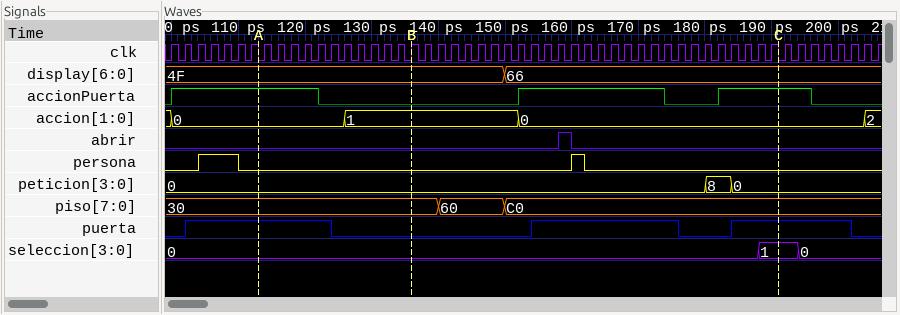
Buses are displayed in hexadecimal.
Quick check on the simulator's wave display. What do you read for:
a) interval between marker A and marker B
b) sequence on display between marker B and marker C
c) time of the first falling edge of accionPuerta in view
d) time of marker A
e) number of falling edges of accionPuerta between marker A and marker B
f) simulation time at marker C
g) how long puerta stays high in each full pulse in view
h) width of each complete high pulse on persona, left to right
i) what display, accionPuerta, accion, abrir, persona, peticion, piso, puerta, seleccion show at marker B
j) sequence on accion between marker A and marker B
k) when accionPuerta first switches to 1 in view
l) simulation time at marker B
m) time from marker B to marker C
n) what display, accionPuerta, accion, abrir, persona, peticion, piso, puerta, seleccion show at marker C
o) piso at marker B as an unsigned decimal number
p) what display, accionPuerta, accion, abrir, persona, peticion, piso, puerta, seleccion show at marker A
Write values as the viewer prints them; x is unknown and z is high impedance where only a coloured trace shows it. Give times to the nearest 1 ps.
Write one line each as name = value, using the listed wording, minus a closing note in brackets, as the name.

interval between marker A and marker B = 23 ps
sequence on display between marker B and marker C = 4F, 66
time of the first falling edge of accionPuerta in view = 122 ps
time of marker A = 113 ps
number of falling edges of accionPuerta between marker A and marker B = 1
simulation time at marker C = 191 ps
how long puerta stays high in each full pulse in view = 22 ps, 22 ps, 18 ps
width of each complete high pulse on persona, left to right = 6 ps, 2 ps
what display, accionPuerta, accion, abrir, persona, peticion, piso, puerta, seleccion show at marker B = display=4F, accionPuerta=0, accion=1, abrir=0, persona=0, peticion=0, piso=30, puerta=0, seleccion=0
sequence on accion between marker A and marker B = 0, 1
when accionPuerta first switches to 1 in view = 100 ps
simulation time at marker B = 136 ps
time from marker B to marker C = 55 ps
what display, accionPuerta, accion, abrir, persona, peticion, piso, puerta, seleccion show at marker C = display=66, accionPuerta=1, accion=0, abrir=0, persona=0, peticion=0, piso=C0, puerta=1, seleccion=1
piso at marker B as an unsigned decimal number = 48
what display, accionPuerta, accion, abrir, persona, peticion, piso, puerta, seleccion show at marker A = display=4F, accionPuerta=1, accion=0, abrir=0, persona=0, peticion=0, piso=30, puerta=1, seleccion=0
